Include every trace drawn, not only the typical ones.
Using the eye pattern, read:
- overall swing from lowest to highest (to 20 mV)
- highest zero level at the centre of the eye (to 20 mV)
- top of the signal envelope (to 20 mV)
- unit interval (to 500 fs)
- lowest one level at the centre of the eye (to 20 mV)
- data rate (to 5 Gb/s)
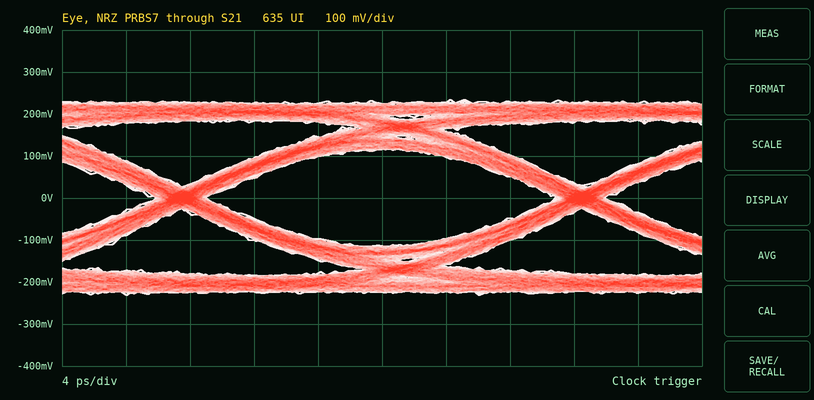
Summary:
460 mV
-120 mV
240 mV
25.0 ps
120 mV
40 Gb/s
